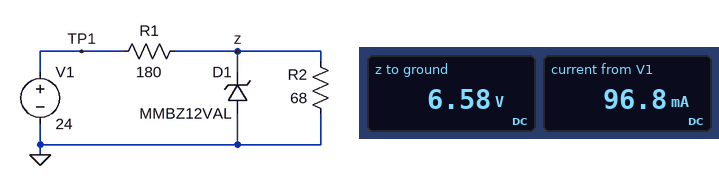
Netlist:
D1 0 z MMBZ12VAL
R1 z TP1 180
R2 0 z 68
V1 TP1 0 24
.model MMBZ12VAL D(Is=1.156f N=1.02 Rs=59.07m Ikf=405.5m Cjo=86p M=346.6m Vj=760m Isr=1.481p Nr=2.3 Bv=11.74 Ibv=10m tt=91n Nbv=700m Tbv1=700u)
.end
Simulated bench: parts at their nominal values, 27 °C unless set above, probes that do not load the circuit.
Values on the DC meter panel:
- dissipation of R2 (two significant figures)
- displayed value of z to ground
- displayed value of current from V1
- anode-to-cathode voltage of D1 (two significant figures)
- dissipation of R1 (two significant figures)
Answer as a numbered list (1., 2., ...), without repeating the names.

1. 640 mW
2. 6.58 V
3. 96.8 mA
4. -6.6 V
5. 1.7 W
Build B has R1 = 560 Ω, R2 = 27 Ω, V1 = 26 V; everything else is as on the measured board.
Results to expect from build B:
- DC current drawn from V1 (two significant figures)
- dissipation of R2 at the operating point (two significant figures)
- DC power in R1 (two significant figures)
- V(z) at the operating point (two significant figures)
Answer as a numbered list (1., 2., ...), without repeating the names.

1. 44 mA
2. 53 mW
3. 1.1 W
4. 1.2 V
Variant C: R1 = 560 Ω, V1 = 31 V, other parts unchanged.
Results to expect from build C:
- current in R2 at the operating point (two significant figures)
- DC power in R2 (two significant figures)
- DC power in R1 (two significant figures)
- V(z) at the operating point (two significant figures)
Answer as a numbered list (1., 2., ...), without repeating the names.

1. 49 mA
2. 170 mW
3. 1.4 W
4. 3.4 V
